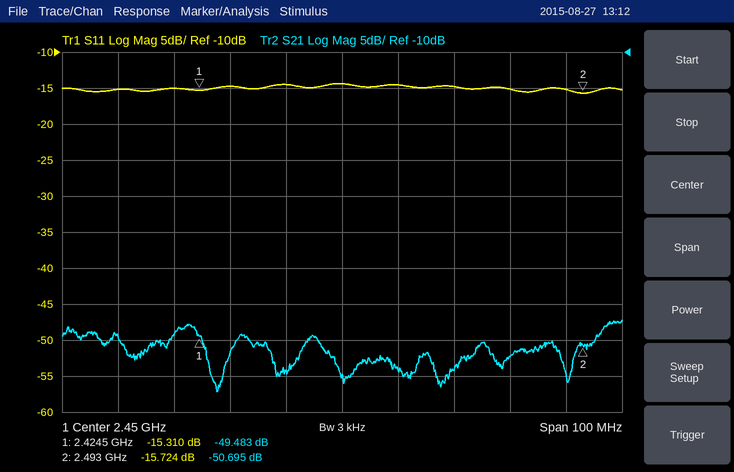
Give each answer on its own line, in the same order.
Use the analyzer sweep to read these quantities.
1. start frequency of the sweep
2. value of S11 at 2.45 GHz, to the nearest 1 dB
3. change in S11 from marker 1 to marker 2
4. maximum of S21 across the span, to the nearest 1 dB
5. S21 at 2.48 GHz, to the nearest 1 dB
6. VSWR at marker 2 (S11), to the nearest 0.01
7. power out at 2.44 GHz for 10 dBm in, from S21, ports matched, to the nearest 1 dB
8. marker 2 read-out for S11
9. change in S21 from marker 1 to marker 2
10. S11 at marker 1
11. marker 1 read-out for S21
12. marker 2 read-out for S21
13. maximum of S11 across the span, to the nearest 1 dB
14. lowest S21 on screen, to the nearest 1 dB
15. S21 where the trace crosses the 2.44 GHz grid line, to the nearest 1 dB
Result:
2.4 GHz
-14 dB
-0.414 dB
-47 dB
-52 dB
1.39
-44 dBm
-15.724 dB
-1.212 dB
-15.310 dB
-49.483 dB
-50.695 dB
-14 dB
-57 dB
-54 dB
